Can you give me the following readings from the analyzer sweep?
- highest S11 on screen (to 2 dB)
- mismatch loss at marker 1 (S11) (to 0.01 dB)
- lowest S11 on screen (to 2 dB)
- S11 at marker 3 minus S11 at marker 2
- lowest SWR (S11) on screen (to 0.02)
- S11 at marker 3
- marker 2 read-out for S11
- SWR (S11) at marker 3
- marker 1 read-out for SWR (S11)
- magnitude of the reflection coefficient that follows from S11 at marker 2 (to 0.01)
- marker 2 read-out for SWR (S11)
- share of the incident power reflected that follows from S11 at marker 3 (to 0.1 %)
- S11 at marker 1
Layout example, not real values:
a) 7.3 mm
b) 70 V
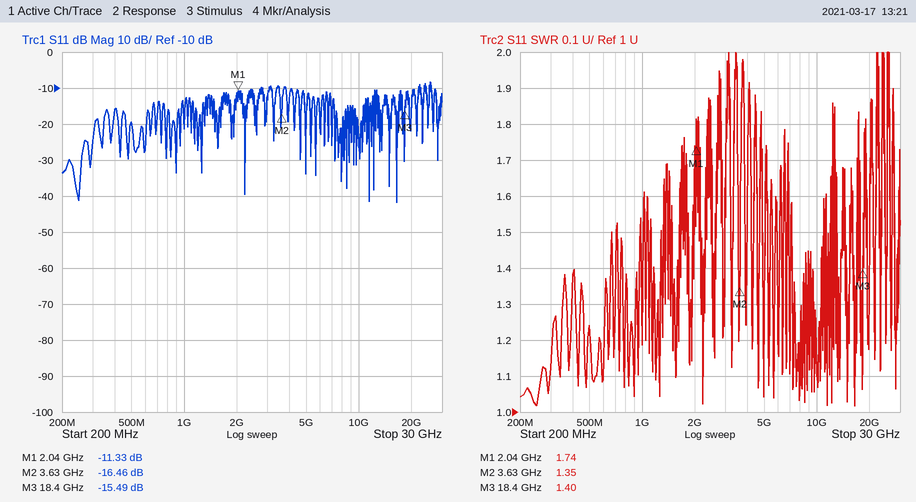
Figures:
a) -8 dB
b) 0.33 dB
c) -42 dB
d) 0.97 dB
e) 1.02
f) -15.49 dB
g) -16.46 dB
h) 1.40
i) 1.74
j) 0.15
k) 1.35
l) 2.8 %
m) -11.33 dB
